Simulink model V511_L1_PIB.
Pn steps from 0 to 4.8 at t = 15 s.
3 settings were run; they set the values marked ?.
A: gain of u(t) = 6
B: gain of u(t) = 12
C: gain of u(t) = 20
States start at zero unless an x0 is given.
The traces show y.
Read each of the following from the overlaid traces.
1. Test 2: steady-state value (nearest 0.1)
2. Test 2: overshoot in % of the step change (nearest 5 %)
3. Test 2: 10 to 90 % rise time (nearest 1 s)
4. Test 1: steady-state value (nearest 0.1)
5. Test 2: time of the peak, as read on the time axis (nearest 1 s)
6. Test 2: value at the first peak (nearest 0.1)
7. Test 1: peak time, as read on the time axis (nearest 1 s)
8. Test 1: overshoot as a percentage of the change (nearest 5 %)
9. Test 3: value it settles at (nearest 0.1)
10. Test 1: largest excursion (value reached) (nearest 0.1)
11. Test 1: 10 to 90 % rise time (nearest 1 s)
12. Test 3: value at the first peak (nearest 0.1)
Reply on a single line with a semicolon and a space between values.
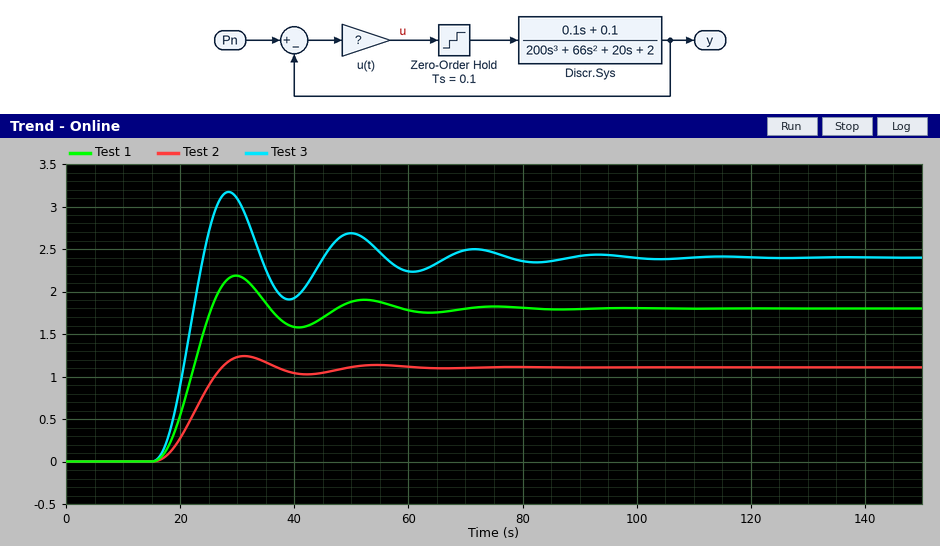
1.1; 10 %; 8 s; 1.8; 31 s; 1.2; 30 s; 20 %; 2.4; 2.2; 7 s; 3.2
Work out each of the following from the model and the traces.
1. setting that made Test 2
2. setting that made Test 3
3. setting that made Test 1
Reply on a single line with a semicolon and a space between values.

A; C; B
